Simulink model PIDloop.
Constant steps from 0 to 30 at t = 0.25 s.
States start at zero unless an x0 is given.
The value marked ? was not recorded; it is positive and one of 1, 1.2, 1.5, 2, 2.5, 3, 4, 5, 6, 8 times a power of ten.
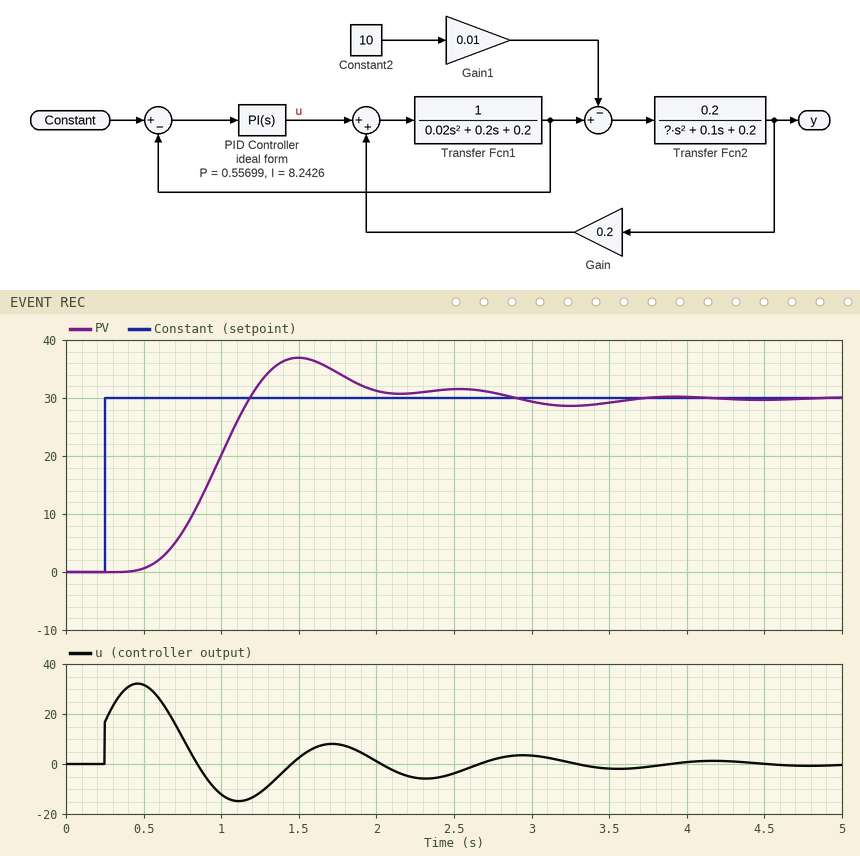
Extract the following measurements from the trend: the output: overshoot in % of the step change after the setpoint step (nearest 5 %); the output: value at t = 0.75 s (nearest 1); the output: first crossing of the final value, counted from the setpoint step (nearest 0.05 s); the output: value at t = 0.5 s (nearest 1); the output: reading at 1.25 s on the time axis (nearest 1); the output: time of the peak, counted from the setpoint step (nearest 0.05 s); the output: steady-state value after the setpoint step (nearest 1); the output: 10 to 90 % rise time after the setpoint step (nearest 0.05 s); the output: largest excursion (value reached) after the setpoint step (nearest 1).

25 %
7
0.95 s
1
33
1.25 s
30
0.50 s
37
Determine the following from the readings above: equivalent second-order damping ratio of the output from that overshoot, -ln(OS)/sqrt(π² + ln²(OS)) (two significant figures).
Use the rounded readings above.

0.40
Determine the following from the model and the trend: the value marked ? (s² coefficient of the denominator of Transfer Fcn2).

0.03
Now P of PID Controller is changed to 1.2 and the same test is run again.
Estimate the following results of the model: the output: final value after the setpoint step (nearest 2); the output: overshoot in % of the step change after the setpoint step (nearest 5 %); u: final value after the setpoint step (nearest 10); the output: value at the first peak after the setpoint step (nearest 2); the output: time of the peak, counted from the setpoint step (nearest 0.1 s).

30
15 %
0
34
1.6 s
